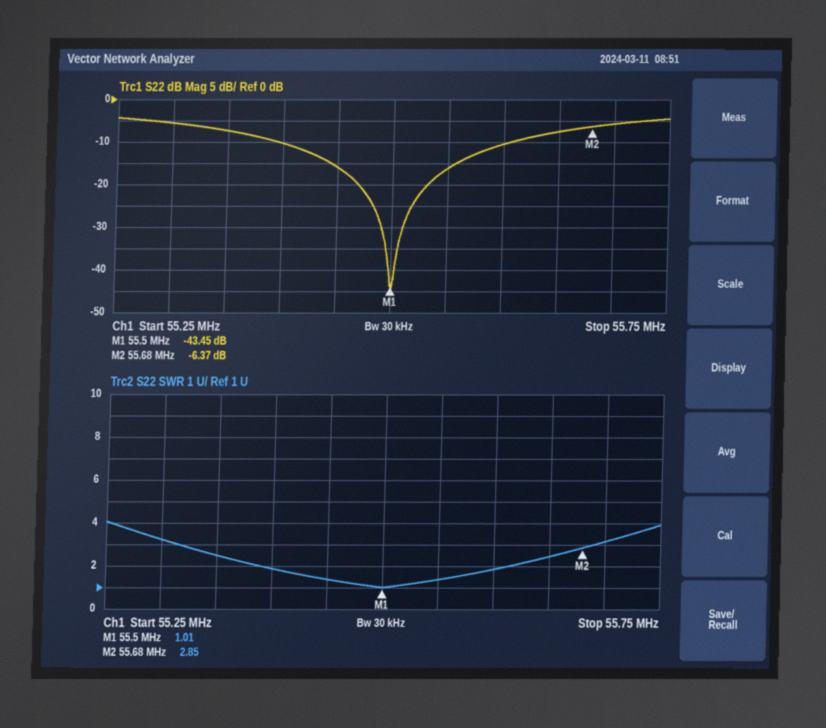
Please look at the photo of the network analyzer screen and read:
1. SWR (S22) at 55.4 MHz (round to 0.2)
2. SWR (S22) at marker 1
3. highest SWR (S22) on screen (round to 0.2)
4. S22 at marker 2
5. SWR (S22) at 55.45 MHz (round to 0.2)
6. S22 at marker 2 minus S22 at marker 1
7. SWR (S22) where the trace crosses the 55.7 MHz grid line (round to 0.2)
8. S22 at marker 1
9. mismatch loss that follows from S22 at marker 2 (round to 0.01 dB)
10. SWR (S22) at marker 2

1.8
1.01
4.0
-6.37 dB
1.4
37.08 dB
3.2
-43.45 dB
1.14 dB
2.85
